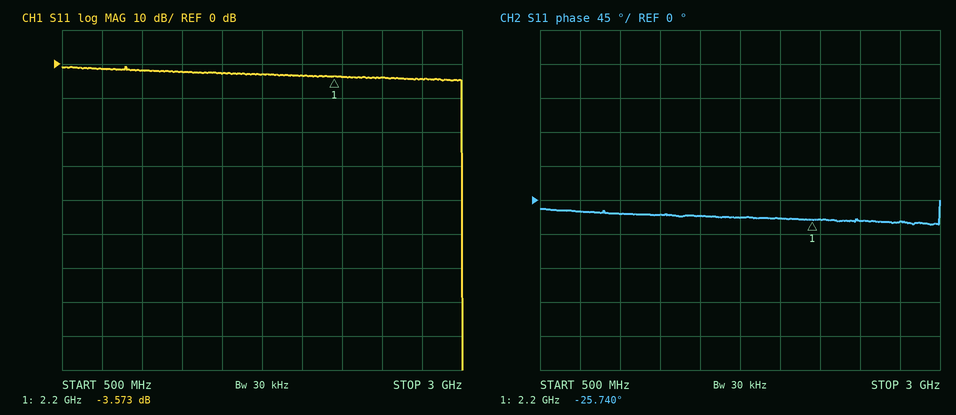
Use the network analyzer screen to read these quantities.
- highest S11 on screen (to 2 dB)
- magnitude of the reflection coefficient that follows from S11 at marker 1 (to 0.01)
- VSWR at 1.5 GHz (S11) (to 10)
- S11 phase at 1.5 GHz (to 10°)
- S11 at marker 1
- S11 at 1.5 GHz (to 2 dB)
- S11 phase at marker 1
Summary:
0 dB
0.66
10
-20°
-3.573 dB
-2 dB
-25.740°
